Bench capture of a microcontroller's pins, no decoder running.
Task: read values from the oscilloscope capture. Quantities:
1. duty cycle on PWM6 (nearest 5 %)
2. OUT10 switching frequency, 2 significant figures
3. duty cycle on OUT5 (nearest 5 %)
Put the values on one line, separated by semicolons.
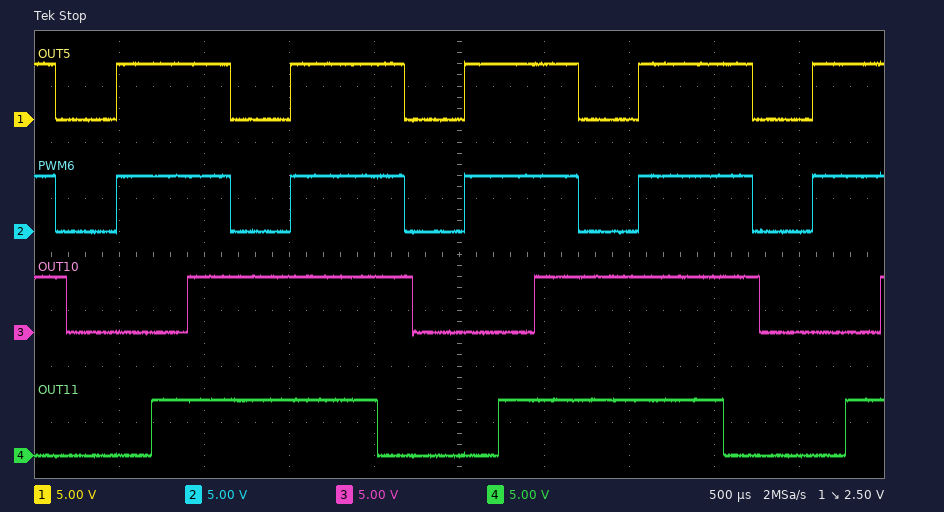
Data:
65 %; 490 Hz; 65 %
